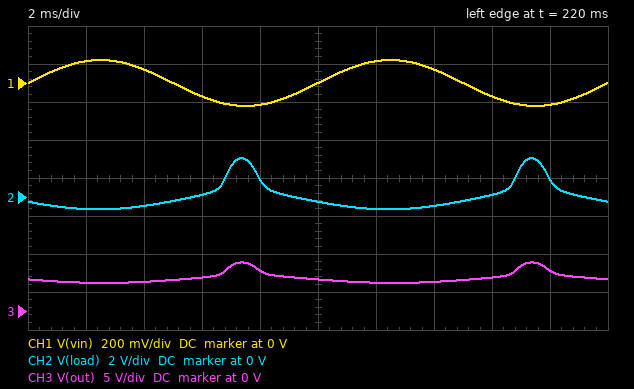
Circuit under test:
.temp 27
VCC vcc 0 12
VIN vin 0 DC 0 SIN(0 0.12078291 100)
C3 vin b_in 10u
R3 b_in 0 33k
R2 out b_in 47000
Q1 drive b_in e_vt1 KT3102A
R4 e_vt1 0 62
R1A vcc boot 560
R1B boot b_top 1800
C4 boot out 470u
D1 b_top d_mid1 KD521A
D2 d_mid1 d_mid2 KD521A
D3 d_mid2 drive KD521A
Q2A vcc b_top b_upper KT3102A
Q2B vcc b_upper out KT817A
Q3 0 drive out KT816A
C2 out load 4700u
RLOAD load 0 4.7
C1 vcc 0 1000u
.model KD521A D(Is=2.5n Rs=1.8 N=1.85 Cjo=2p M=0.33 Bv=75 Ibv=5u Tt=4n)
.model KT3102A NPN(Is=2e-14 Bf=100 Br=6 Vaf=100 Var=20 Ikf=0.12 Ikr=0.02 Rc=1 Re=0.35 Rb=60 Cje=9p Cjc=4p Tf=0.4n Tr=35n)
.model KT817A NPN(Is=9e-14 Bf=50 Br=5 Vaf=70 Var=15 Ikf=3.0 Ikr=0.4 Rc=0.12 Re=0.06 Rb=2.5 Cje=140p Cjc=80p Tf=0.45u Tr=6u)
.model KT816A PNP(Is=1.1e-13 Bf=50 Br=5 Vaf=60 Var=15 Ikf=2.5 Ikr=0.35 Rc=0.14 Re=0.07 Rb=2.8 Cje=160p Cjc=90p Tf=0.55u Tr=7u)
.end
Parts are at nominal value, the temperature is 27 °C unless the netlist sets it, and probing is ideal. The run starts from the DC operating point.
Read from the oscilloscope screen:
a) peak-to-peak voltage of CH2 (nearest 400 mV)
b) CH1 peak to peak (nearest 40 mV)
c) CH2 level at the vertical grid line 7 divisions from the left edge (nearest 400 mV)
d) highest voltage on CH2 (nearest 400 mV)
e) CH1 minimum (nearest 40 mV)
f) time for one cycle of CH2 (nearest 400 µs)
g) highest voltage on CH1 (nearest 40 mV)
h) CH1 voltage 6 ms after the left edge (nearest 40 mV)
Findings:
2.8 V
240 mV
-400 mV
2.0 V
-120 mV
10.0 ms
120 mV
-80 mV
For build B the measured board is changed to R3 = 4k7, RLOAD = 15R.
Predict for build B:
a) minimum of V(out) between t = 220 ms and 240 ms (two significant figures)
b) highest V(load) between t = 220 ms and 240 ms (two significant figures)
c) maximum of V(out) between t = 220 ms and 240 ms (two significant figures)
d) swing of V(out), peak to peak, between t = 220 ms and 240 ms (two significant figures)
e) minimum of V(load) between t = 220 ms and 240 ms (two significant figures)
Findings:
7.3 V
2.3 V
11 V
4.0 V
-1.7 V
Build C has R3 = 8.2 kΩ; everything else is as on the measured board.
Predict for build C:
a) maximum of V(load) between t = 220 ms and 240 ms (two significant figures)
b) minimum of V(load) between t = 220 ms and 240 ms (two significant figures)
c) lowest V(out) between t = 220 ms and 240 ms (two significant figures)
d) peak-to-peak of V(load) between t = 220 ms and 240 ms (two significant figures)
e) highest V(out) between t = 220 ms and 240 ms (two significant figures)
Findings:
2.3 V
-680 mV
6.4 V
3.0 V
9.4 V
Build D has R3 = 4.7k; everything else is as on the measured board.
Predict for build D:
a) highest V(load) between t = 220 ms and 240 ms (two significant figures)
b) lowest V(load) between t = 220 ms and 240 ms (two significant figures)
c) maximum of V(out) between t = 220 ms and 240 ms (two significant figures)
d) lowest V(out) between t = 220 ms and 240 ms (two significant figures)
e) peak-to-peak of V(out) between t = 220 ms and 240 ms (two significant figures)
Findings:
1.8 V
-640 mV
11 V
8.6 V
2.4 V
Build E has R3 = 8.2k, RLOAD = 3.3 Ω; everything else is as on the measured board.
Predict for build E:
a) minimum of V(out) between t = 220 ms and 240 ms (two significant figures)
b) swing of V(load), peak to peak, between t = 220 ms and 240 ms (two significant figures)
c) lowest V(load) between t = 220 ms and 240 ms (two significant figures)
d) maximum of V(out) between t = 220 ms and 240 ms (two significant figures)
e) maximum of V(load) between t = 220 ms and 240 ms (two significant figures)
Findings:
6.6 V
2.1 V
-480 mV
8.7 V
1.6 V
